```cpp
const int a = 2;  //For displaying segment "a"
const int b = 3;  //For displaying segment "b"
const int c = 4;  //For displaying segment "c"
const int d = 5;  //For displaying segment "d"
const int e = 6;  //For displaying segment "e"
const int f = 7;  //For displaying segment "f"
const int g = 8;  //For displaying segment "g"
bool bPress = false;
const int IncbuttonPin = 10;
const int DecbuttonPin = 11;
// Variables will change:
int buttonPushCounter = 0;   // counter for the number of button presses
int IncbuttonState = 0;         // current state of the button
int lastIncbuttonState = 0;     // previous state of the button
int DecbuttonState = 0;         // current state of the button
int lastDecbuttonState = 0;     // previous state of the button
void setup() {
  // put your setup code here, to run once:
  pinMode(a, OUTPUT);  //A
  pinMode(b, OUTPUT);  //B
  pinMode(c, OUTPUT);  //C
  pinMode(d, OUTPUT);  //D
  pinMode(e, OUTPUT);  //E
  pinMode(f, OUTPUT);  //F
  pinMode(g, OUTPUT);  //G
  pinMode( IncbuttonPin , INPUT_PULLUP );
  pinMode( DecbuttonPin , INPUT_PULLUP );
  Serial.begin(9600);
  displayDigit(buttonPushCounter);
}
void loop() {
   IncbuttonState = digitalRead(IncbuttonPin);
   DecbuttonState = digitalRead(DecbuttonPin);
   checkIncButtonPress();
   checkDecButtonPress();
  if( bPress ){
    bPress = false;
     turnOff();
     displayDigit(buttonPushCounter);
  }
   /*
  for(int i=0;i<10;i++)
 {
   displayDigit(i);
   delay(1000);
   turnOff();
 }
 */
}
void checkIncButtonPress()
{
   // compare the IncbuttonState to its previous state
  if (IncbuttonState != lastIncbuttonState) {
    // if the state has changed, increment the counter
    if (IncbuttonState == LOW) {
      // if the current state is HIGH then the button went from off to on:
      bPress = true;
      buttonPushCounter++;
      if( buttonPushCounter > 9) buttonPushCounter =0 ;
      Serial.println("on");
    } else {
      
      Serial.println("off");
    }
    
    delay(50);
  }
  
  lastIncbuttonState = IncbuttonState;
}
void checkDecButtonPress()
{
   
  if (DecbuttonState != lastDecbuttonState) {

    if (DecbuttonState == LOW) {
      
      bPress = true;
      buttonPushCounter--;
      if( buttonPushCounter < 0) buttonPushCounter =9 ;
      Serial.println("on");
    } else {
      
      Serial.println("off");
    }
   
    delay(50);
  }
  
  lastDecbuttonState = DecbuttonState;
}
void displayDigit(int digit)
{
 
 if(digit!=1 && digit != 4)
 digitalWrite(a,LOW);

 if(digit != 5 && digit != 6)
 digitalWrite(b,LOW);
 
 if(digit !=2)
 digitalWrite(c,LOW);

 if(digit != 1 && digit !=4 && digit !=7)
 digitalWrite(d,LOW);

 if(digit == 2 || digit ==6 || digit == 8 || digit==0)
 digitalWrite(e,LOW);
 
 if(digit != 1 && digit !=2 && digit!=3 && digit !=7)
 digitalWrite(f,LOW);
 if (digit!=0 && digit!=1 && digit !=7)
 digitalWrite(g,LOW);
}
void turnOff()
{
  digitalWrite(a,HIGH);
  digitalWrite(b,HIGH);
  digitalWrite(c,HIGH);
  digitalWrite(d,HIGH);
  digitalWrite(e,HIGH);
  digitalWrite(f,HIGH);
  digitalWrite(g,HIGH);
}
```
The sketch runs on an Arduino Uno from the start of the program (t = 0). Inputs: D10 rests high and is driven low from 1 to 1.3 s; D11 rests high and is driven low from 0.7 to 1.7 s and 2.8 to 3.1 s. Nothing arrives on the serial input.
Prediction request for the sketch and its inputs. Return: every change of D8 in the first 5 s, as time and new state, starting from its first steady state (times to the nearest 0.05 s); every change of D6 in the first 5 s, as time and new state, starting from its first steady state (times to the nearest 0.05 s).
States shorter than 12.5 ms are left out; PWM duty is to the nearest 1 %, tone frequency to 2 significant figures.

0 s low; 1.05 s high; 2.85 s low
0 s low; 0.75 s high; 1.05 s low; 2.85 s high
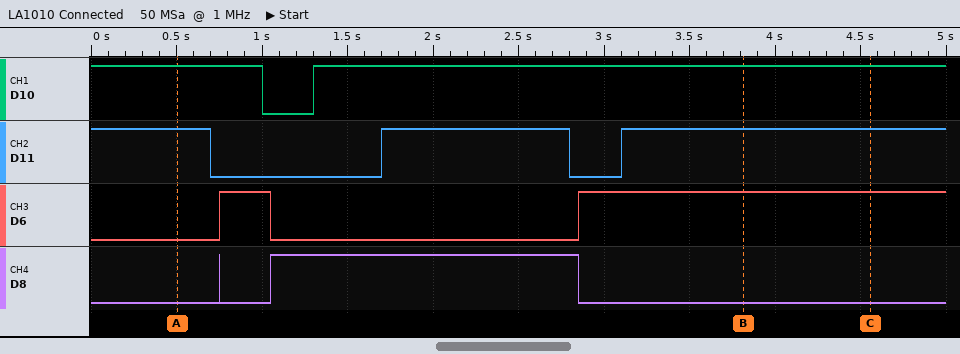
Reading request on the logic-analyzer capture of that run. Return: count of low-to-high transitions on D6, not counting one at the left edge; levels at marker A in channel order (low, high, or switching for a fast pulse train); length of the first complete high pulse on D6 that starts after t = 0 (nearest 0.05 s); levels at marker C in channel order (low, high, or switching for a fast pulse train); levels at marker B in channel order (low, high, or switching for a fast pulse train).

2
D10 high, D11 high, D6 low, D8 low
0.30 s
D10 high, D11 high, D6 high, D8 low
D10 high, D11 high, D6 high, D8 low
